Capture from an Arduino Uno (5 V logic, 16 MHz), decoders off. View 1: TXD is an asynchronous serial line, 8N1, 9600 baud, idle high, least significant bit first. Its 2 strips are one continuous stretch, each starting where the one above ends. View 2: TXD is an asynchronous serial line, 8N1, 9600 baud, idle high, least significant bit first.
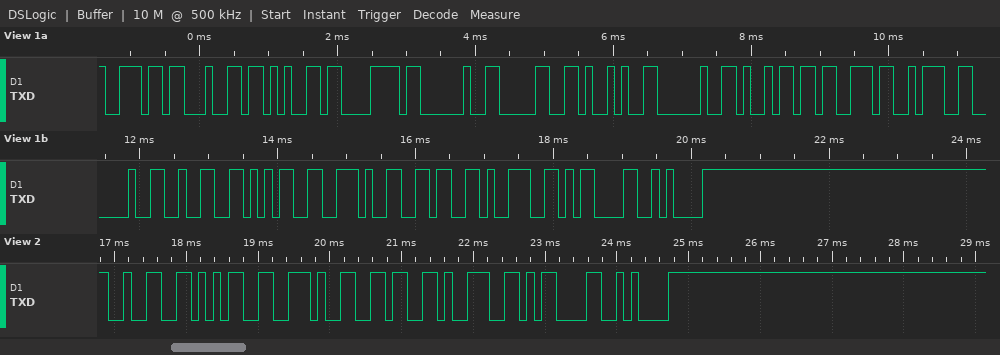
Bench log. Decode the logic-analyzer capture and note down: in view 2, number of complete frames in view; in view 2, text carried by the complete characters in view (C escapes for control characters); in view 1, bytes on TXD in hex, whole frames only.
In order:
7
"25.69\r\n"
6E 64 65 78 20 30 29 20 69 73 3A 20 32 35 2E 36 39 0D 0A
